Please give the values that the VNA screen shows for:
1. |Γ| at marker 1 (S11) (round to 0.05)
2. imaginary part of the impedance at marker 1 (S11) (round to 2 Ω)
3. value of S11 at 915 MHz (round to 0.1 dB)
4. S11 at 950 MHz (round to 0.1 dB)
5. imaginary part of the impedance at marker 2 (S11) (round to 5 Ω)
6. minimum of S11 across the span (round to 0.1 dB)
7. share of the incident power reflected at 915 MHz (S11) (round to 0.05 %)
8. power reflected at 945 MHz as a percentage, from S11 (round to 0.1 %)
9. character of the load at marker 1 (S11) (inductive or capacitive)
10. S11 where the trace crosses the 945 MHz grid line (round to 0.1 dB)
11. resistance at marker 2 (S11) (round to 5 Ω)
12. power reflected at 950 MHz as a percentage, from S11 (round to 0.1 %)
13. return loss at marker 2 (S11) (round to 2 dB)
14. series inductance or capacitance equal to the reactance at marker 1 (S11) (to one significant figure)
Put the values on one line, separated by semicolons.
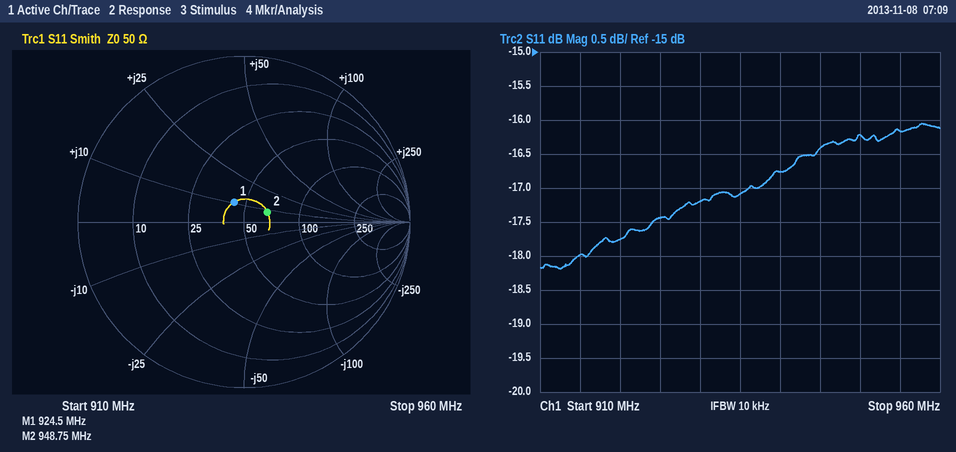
0.15; +10 Ω; -18.0 dB; -16.2 dB; +10 Ω; -18.2 dB; 1.60 %; 2.3 %; inductive; -16.4 dB; 65 Ω; 2.4 %; 16 dB; 2 nH
